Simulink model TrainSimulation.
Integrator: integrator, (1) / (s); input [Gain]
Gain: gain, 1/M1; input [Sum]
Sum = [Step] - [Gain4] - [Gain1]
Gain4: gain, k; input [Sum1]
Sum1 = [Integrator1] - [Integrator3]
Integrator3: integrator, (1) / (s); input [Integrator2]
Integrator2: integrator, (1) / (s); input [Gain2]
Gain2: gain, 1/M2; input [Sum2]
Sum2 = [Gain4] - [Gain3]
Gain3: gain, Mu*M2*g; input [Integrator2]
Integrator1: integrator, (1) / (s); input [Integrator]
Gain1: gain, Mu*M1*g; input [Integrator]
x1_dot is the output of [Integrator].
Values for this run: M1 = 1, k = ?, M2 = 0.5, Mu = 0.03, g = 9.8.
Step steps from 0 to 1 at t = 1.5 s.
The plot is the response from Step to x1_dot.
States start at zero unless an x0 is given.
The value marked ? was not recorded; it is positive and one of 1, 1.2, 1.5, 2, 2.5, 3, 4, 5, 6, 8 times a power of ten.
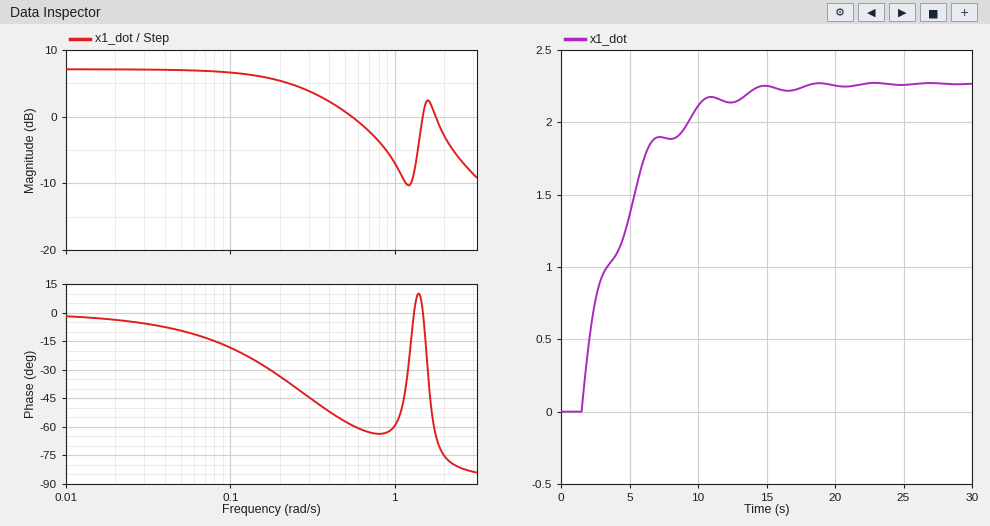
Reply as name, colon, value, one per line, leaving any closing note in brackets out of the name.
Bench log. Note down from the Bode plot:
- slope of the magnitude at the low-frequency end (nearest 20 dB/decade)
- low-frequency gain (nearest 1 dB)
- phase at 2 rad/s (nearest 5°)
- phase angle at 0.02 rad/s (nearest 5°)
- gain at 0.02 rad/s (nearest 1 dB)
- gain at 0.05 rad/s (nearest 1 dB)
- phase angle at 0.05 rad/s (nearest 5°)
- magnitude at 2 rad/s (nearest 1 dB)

slope of the magnitude at the low-frequency end: 0 dB/decade
low-frequency gain: 7 dB
phase at 2 rad/s: -75°
phase angle at 0.02 rad/s: -5°
gain at 0.02 rad/s: 7 dB
gain at 0.05 rad/s: 7 dB
phase angle at 0.05 rad/s: -10°
magnitude at 2 rad/s: -3 dB
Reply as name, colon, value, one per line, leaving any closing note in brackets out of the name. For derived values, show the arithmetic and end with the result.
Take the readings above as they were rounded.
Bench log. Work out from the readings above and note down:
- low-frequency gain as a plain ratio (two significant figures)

low-frequency gain as a plain ratio: 10^(7 / 20) = 2.2
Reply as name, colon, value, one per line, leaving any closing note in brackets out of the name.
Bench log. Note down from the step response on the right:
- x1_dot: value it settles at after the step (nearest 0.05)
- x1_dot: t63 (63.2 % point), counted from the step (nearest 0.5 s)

x1_dot: value it settles at after the step: 2.25
x1_dot: t63 (63.2 % point), counted from the step: 3.5 s
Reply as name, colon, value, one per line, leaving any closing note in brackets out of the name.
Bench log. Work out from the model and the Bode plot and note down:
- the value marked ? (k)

the value marked ?: 0.8
